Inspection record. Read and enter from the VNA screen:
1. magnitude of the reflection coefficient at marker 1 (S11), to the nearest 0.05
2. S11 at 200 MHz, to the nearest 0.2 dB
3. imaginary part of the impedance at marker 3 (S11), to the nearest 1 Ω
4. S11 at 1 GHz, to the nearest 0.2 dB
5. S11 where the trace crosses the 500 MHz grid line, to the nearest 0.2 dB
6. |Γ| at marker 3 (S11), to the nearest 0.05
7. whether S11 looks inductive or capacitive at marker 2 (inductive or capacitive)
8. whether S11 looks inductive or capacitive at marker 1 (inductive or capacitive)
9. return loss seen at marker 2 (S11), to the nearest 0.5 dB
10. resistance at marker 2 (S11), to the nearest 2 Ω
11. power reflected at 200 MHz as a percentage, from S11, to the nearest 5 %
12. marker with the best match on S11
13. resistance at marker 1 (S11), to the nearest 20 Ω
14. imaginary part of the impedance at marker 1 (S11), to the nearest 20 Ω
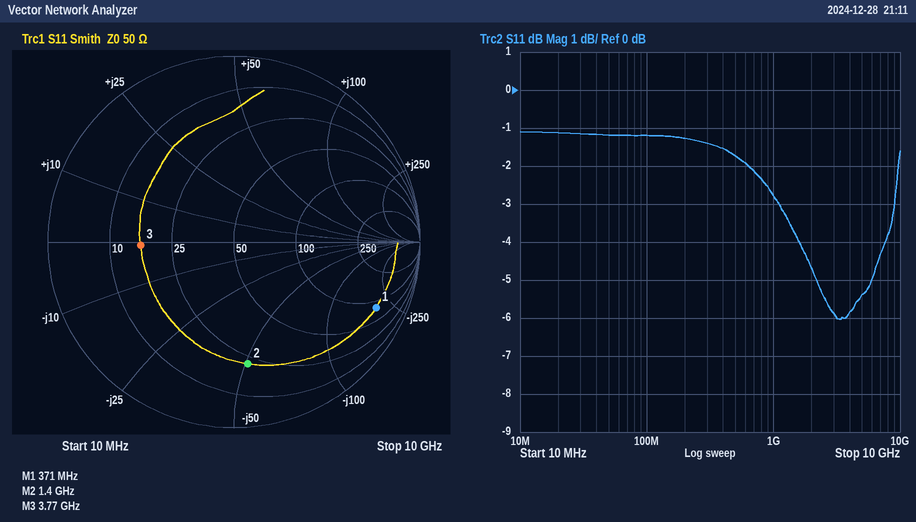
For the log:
0.85
-1.2 dB
-1 Ω
-2.8 dB
-1.8 dB
0.50
capacitive
capacitive
3.5 dB
22 Ω
75 %
marker 3
80 Ω
-200 Ω
